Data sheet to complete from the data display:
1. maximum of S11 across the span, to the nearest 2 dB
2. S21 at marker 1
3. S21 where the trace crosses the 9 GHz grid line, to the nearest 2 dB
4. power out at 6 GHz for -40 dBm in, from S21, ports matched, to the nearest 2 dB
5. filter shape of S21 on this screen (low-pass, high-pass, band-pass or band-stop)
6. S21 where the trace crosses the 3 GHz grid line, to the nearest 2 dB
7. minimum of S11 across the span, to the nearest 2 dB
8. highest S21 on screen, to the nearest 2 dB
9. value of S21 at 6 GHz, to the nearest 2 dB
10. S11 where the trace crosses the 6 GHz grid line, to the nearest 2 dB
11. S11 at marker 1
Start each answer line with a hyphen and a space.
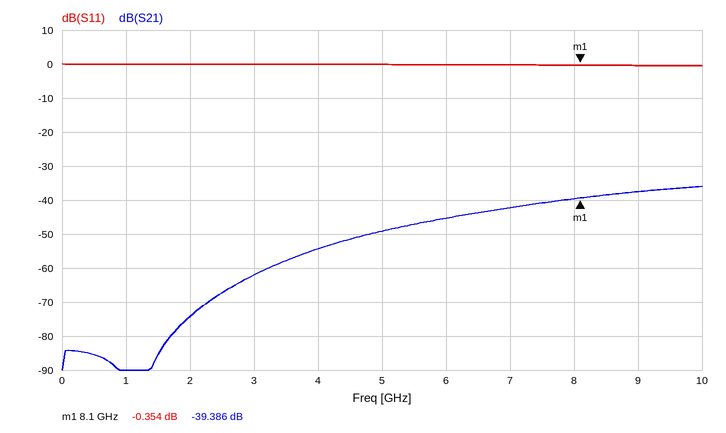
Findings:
- 0 dB
- -39.386 dB
- -38 dB
- -86 dBm
- high-pass
- -62 dB
- 0 dB
- -36 dB
- -46 dB
- 0 dB
- -0.354 dB
